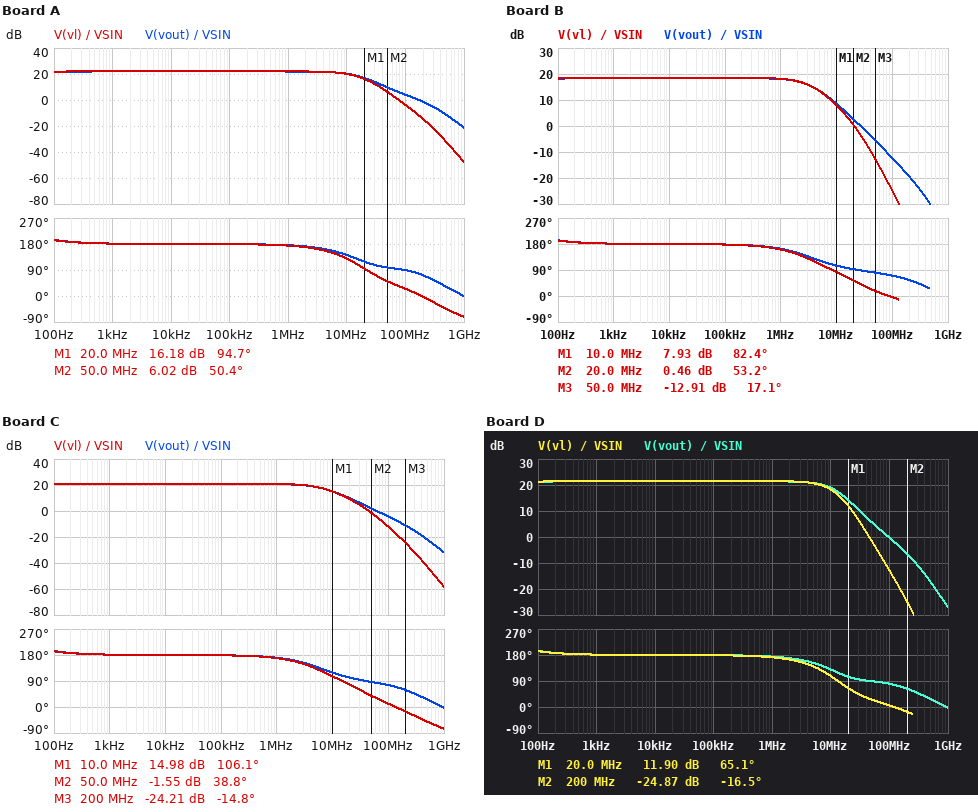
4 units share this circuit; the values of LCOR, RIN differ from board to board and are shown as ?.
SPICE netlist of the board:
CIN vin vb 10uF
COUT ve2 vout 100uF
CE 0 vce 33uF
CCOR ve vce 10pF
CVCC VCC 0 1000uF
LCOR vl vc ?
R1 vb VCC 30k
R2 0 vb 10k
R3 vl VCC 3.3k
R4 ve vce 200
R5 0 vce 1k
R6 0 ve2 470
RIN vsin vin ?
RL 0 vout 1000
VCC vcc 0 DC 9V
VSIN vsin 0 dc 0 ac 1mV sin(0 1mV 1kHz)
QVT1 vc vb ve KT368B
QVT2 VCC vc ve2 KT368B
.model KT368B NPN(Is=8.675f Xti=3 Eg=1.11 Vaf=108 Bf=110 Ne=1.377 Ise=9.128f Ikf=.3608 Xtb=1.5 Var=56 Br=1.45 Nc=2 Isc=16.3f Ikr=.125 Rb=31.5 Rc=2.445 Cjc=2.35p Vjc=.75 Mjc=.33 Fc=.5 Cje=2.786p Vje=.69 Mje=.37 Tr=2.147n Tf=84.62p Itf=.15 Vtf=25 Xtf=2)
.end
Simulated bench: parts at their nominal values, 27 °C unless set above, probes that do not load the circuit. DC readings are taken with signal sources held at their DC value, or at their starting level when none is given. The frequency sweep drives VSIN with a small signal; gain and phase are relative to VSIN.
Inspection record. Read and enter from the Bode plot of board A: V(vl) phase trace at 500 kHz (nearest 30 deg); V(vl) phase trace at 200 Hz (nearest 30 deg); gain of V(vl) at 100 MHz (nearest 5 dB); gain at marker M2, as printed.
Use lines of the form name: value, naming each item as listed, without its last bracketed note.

V(vl) phase trace at 500 kHz: 180 deg
V(vl) phase trace at 200 Hz: 180 deg
gain of V(vl) at 100 MHz: -5 dB
gain at marker M2, as printed: 6.02 dB
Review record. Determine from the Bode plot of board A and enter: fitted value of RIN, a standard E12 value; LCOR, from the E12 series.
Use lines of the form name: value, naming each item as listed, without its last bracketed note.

fitted value of RIN, a standard E12 value: 330 Ω
LCOR, from the E12 series: 12 µH
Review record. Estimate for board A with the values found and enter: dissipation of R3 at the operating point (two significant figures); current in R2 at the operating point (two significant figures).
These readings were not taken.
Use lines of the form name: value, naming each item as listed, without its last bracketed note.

dissipation of R3 at the operating point: 5.7 mW
current in R2 at the operating point: 220 µA
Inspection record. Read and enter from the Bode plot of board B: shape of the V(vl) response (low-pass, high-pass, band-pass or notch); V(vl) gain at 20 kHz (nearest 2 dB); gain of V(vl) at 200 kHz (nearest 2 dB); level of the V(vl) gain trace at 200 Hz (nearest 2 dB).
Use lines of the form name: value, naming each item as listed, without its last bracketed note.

shape of the V(vl) response: low-pass
V(vl) gain at 20 kHz: 18 dB
gain of V(vl) at 200 kHz: 18 dB
level of the V(vl) gain trace at 200 Hz: 18 dB
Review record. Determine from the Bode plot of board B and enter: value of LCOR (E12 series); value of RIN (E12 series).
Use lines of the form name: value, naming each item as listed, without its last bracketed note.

value of LCOR: 22 µH
value of RIN: 3.3 kΩ
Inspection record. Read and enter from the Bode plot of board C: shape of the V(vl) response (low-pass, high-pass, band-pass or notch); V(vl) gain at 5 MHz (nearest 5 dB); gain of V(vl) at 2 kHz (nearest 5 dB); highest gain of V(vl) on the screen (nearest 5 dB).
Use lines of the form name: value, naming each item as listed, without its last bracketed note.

shape of the V(vl) response: low-pass
V(vl) gain at 5 MHz: 20 dB
gain of V(vl) at 2 kHz: 20 dB
highest gain of V(vl) on the screen: 20 dB
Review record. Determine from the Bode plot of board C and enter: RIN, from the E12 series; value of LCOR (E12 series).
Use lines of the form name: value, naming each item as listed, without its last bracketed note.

RIN, from the E12 series: 1.2 kΩ
value of LCOR: 12 µH
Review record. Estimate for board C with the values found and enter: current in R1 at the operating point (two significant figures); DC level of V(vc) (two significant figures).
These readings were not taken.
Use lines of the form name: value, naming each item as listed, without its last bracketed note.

current in R1 at the operating point: 230 µA
DC level of V(vc): 4.7 V
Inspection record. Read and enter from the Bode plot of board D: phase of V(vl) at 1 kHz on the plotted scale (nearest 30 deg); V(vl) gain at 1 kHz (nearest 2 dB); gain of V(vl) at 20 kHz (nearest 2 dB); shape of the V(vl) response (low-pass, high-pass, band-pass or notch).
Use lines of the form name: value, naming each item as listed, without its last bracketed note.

phase of V(vl) at 1 kHz on the plotted scale: 180 deg
V(vl) gain at 1 kHz: 22 dB
gain of V(vl) at 20 kHz: 22 dB
shape of the V(vl) response: low-pass
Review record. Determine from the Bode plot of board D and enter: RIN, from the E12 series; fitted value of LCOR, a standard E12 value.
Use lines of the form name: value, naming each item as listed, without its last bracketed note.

RIN, from the E12 series: 680 Ω
fitted value of LCOR, a standard E12 value: 22 µH
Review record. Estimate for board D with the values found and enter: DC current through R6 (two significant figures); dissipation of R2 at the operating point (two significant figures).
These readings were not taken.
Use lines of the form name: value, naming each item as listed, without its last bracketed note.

DC current through R6: 8.4 mA
dissipation of R2 at the operating point: 470 µW
